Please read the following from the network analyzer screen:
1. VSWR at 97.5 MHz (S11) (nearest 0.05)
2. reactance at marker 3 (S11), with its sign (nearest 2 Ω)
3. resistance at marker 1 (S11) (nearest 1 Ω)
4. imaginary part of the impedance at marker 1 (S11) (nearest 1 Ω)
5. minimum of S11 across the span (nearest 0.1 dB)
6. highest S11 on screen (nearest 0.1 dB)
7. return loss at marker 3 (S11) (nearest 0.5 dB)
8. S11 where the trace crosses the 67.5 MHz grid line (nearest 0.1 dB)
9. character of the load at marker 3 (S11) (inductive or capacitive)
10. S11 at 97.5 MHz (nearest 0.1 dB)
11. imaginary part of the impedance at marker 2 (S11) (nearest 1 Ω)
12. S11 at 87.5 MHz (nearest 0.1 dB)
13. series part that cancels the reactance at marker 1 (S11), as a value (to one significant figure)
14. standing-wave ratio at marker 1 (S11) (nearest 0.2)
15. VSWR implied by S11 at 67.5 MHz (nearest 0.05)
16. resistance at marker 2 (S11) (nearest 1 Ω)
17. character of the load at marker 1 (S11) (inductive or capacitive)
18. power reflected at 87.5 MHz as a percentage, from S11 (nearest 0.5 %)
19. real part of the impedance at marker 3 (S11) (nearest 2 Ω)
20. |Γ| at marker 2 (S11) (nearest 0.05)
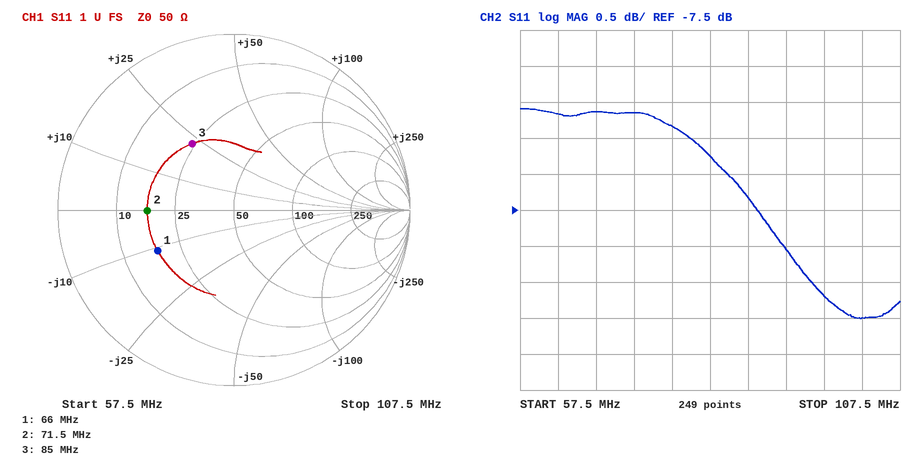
2.15
+22 Ω
18 Ω
-11 Ω
-9.0 dB
-6.1 dB
7.0 dB
-6.1 dB
inductive
-8.7 dB
0 Ω
-7.3 dB
30 nH
3.0
2.95
17 Ω
capacitive
18.5 %
24 Ω
0.50
